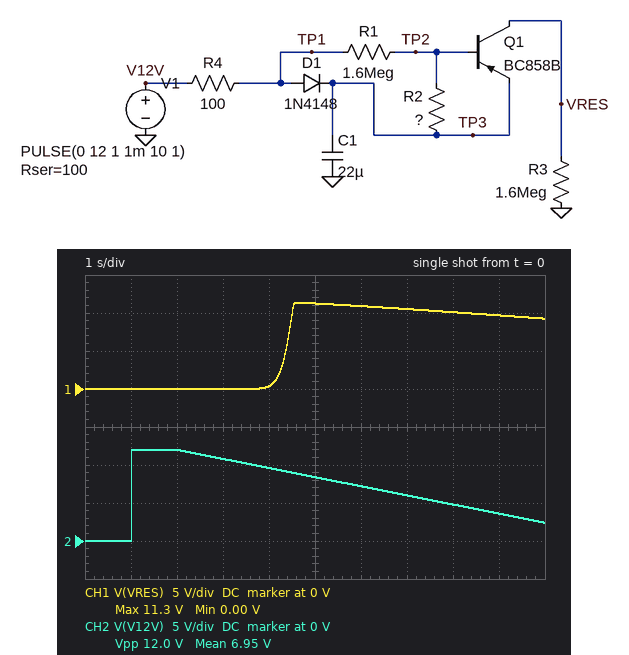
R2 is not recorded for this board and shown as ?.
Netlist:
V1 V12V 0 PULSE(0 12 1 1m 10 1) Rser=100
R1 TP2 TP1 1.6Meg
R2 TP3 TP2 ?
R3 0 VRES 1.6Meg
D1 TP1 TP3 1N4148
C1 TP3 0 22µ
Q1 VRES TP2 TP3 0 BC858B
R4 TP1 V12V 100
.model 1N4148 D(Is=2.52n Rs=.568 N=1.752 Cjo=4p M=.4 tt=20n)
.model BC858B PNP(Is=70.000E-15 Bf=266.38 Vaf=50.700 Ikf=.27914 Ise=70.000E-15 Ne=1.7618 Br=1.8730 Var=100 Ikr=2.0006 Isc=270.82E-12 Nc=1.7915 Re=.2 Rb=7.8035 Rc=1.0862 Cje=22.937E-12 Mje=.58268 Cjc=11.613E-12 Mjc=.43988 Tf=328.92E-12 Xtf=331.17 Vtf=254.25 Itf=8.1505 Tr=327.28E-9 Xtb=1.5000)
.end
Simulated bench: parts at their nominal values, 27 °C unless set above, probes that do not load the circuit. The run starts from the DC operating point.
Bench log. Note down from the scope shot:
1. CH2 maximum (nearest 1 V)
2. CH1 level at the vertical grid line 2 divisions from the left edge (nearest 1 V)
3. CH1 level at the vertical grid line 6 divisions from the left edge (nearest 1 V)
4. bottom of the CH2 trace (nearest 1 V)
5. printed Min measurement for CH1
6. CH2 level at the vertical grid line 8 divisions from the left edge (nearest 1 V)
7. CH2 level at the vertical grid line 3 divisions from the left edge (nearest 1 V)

12 V
0 V
11 V
0 V
0.00 V
5 V
11 V
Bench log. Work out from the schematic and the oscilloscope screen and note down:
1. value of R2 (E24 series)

360 kΩ
